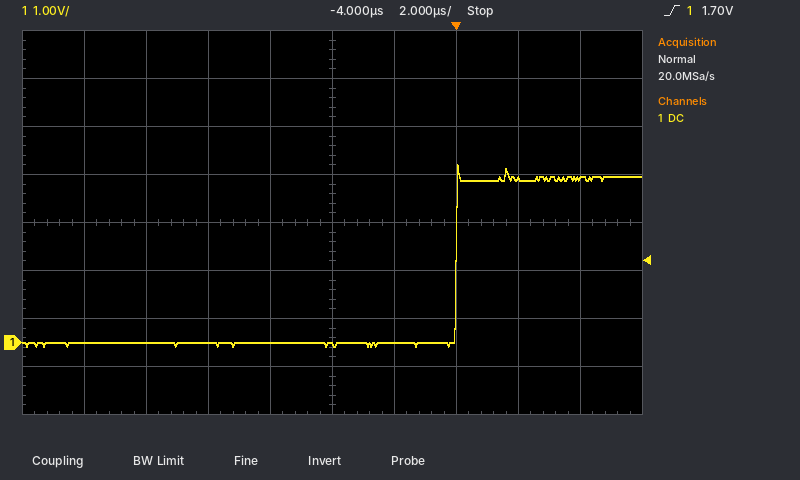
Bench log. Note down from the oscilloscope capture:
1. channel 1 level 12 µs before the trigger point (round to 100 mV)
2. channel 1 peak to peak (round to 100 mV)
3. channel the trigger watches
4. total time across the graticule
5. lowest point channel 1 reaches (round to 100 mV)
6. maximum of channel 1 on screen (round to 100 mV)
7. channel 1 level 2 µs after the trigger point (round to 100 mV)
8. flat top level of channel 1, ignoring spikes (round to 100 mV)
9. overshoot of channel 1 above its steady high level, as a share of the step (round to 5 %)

0.0 V
3.8 V
channel 1
20 µs
-100 mV
3.7 V
3.4 V
3.4 V
10 %
